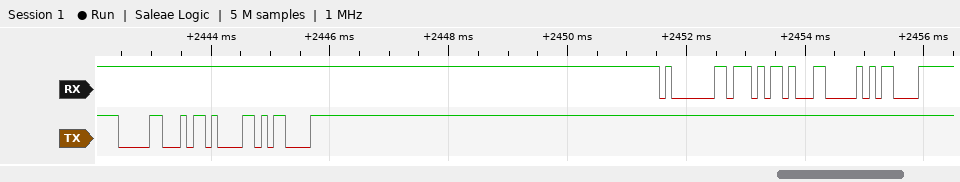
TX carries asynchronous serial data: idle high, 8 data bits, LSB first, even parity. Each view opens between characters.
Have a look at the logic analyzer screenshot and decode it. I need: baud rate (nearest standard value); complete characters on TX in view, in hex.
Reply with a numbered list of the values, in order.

1. 9600 baud
2. 30, 0B, 0D
